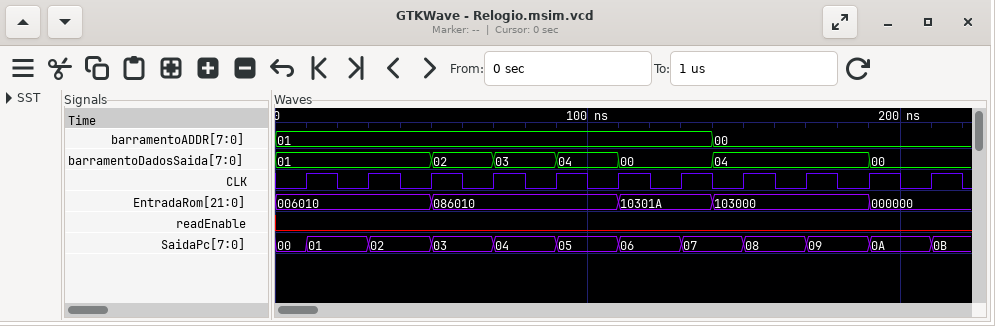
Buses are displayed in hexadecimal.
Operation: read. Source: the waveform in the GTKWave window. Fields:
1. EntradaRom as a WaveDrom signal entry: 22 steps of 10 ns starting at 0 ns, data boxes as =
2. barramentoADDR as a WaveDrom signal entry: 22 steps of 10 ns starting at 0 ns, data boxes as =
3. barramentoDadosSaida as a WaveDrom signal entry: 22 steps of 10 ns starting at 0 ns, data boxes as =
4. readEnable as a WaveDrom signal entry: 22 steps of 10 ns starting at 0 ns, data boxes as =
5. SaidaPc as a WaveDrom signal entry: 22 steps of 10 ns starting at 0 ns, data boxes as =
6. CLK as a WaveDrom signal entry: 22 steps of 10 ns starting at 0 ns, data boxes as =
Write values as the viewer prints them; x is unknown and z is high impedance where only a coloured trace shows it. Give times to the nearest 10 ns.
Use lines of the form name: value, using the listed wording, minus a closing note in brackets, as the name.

EntradaRom as a WaveDrom signal entry: 22 steps of 10 ns starting at 0 ns, data boxes as =: {name: 'EntradaRom', wave: '=....=.....=..=....=..', data: '006010 086010 10301A 103000 000000'}
barramentoADDR as a WaveDrom signal entry: 22 steps of 10 ns starting at 0 ns, data boxes as =: {name: 'barramentoADDR', wave: '=.............=.......', data: '01 00'}
barramentoDadosSaida as a WaveDrom signal entry: 22 steps of 10 ns starting at 0 ns, data boxes as =: {name: 'barramentoDadosSaida', wave: '=....=.=.=.=..=....=..', data: '01 02 03 04 00 04 00'}
readEnable as a WaveDrom signal entry: 22 steps of 10 ns starting at 0 ns, data boxes as =: {name: 'readEnable', wave: '0.....................'}
SaidaPc as a WaveDrom signal entry: 22 steps of 10 ns starting at 0 ns, data boxes as =: {name: 'SaidaPc', wave: '==.=.=.=.=.=.=.=.=.=.=', data: '00 01 02 03 04 05 06 07 08 09 0A 0B'}
CLK as a WaveDrom signal entry: 22 steps of 10 ns starting at 0 ns, data boxes as =: {name: 'CLK', wave: '0101010101010101010101'}
